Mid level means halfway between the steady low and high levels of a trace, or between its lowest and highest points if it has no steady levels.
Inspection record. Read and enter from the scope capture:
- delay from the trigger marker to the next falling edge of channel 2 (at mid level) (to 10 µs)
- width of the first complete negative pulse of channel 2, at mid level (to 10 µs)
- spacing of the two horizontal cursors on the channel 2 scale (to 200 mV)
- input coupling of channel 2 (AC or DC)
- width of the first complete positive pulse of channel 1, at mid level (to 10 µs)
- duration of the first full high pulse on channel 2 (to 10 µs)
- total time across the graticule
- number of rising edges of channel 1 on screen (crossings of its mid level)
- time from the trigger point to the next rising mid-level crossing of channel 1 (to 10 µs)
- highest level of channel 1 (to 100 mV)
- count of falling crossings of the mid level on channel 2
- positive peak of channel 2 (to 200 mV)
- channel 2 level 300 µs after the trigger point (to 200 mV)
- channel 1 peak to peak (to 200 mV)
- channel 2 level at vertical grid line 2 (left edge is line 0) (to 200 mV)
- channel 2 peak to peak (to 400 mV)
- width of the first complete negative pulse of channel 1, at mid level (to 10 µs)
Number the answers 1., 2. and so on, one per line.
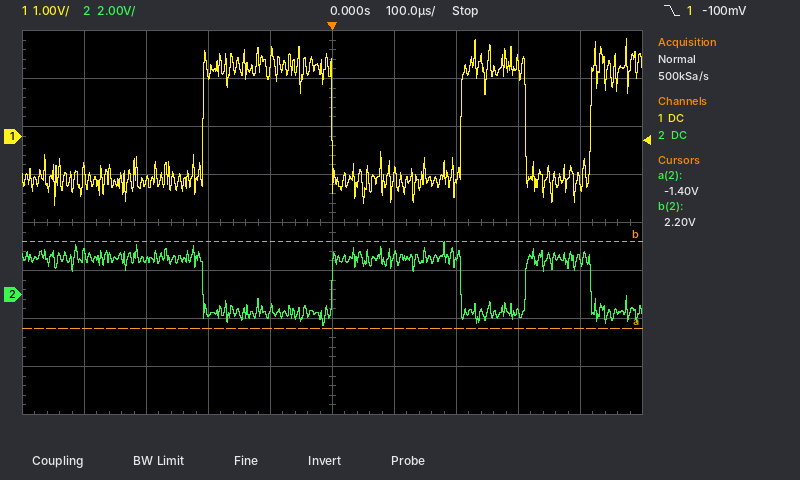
1. 210 µs
2. 210 µs
3. 3.6 V
4. DC
5. 210 µs
6. 210 µs
7. 1 ms
8. 3
9. 210 µs
10. 2.0 V
11. 3
12. 2.2 V
13. -800 mV
14. 3.4 V
15. 1.4 V
16. 3.6 V
17. 210 µs
